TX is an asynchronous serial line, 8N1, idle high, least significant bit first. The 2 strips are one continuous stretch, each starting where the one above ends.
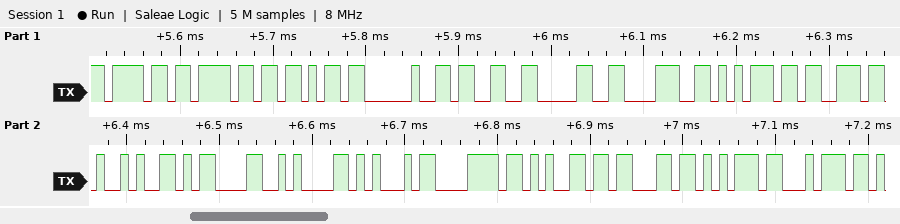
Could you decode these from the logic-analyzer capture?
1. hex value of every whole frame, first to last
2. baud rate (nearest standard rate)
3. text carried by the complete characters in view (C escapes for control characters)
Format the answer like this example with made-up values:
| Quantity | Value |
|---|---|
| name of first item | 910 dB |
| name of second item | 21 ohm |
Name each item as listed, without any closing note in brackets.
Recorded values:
| Quantity | Value |
|---|---|
| hex value of every whole frame, first to last | 6F 6F 6B 20 33 30 38 75 73 29 0D 0A 45 78 65 63 75 74 |
| baud rate | 115200 baud |
| text carried by the complete characters in view | "ook 308us)\r\nExecut" |
